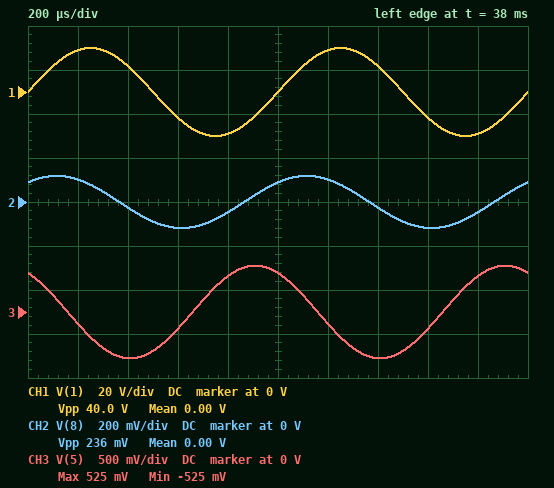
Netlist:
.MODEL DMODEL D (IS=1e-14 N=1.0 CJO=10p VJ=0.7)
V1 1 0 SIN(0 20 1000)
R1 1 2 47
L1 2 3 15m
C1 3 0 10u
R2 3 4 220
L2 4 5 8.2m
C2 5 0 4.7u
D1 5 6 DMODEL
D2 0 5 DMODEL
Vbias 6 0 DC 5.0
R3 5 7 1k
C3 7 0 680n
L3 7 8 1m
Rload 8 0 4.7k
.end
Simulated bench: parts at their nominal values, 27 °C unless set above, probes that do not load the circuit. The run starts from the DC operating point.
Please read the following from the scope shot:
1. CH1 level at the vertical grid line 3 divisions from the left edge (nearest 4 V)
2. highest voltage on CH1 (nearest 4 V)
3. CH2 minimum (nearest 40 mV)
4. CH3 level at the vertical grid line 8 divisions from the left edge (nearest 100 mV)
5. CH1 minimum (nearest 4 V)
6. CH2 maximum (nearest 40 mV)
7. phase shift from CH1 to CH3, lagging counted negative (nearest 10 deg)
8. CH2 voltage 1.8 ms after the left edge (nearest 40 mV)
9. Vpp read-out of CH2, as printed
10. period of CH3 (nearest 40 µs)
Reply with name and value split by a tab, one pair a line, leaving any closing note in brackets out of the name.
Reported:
CH1 level at the vertical grid line 3 divisions from the left edge	-12 V
highest voltage on CH1	20 V
CH2 minimum	-120 mV
CH3 level at the vertical grid line 8 divisions from the left edge	-200 mV
CH1 minimum	-20 V
CH2 maximum	120 mV
phase shift from CH1 to CH3, lagging counted negative	120 deg
CH2 voltage 1.8 ms after the left edge	-40 mV
Vpp read-out of CH2, as printed	236 mV
period of CH3	1.00 ms
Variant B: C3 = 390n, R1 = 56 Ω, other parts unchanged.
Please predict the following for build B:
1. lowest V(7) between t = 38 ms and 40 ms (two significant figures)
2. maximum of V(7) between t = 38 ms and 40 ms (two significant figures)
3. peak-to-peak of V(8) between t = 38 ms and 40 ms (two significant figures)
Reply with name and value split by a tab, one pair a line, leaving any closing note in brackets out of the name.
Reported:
lowest V(7) between t = 38 ms and 40 ms	-180 mV
maximum of V(7) between t = 38 ms and 40 ms	180 mV
peak-to-peak of V(8) between t = 38 ms and 40 ms	360 mV
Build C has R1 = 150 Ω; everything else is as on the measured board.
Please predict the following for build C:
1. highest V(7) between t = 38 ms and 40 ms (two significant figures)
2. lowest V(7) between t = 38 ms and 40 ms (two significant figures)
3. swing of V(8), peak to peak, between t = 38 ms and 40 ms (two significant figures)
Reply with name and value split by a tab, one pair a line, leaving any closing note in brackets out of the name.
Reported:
highest V(7) between t = 38 ms and 40 ms	64 mV
lowest V(7) between t = 38 ms and 40 ms	-64 mV
swing of V(8), peak to peak, between t = 38 ms and 40 ms	130 mV
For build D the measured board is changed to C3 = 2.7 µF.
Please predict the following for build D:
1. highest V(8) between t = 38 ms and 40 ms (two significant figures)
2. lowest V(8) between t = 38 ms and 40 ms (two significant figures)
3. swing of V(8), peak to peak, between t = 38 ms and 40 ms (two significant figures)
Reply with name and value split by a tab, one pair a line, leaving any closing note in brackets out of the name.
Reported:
highest V(8) between t = 38 ms and 40 ms	31 mV
lowest V(8) between t = 38 ms and 40 ms	-31 mV
swing of V(8), peak to peak, between t = 38 ms and 40 ms	62 mV
